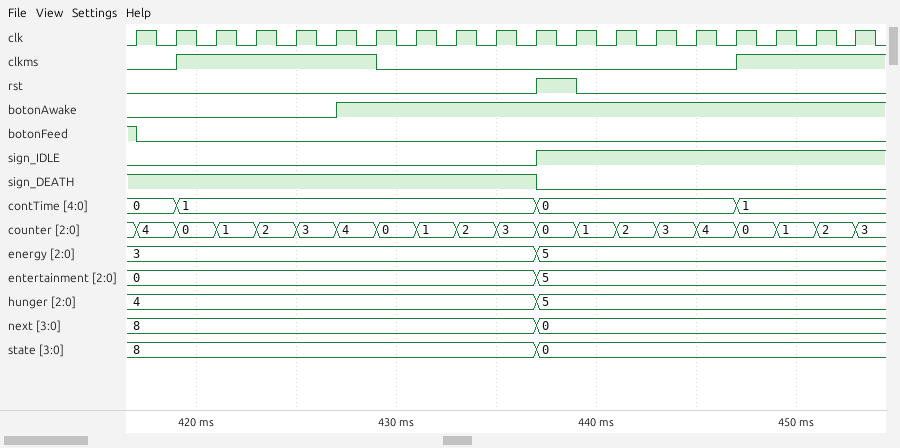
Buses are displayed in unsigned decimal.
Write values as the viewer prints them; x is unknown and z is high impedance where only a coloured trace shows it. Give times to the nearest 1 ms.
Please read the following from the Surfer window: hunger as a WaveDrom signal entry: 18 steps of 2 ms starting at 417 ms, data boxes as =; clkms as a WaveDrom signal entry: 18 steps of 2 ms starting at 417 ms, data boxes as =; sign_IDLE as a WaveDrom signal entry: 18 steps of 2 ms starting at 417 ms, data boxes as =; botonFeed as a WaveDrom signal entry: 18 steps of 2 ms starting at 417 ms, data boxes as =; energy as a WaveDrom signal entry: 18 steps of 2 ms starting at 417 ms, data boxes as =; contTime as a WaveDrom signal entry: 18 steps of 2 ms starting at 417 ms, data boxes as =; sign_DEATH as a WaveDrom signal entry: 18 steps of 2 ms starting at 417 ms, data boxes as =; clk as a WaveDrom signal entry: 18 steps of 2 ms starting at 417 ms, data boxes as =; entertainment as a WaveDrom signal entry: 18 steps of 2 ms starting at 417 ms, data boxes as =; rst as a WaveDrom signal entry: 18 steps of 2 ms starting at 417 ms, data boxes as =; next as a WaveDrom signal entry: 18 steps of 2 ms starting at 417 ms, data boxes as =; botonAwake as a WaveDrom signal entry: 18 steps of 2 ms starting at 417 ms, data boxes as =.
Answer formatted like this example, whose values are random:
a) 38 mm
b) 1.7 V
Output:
a) {name: 'hunger', wave: '=.........=.......', data: '4 5'}
b) {name: 'clkms', wave: '01....0........1..'}
c) {name: 'sign_IDLE', wave: '0.........1.......'}
d) {name: 'botonFeed', wave: '0.................'}
e) {name: 'energy', wave: '=.........=.......', data: '3 5'}
f) {name: 'contTime', wave: '==........=....=..', data: '0 1 0 1'}
g) {name: 'sign_DEATH', wave: '1.........0.......'}
h) {name: 'clk', wave: 'p.................'}
i) {name: 'entertainment', wave: '=.........=.......', data: '0 5'}
j) {name: 'rst', wave: '0.........10......'}
k) {name: 'next', wave: '=.........=.......', data: '8 0'}
l) {name: 'botonAwake', wave: '0....1............'}
